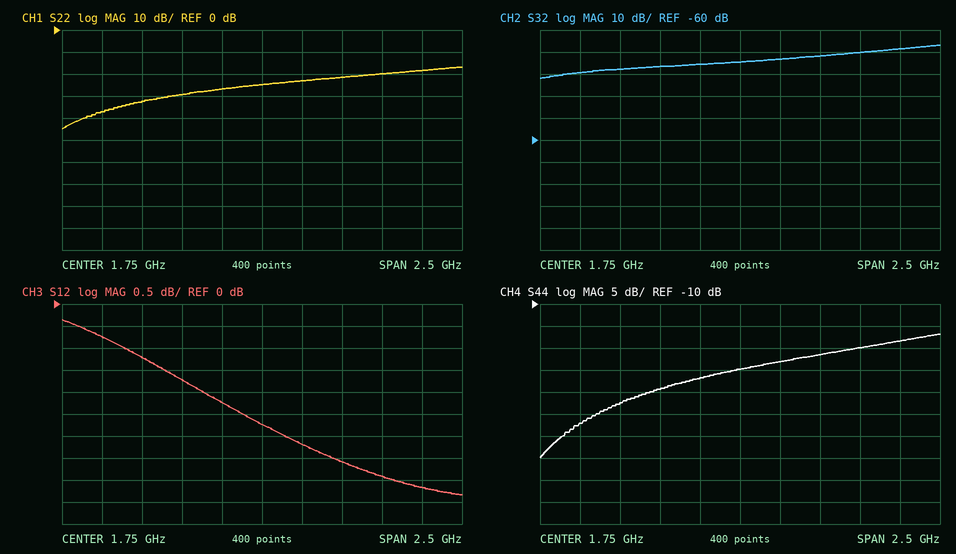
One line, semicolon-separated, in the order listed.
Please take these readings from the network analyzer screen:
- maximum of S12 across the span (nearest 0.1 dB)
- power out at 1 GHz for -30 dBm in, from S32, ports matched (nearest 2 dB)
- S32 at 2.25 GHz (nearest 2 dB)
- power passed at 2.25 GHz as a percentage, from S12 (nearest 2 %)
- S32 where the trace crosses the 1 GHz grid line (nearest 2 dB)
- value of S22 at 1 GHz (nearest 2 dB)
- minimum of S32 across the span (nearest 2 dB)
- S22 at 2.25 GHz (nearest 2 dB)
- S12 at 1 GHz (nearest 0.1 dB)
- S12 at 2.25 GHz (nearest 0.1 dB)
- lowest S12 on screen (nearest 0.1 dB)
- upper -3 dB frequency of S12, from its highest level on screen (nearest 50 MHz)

-0.4 dB; -58 dBm; -22 dB; 44 %; -28 dB; -32 dB; -32 dB; -22 dB; -1.2 dB; -3.6 dB; -4.3 dB; 2.10 GHz
